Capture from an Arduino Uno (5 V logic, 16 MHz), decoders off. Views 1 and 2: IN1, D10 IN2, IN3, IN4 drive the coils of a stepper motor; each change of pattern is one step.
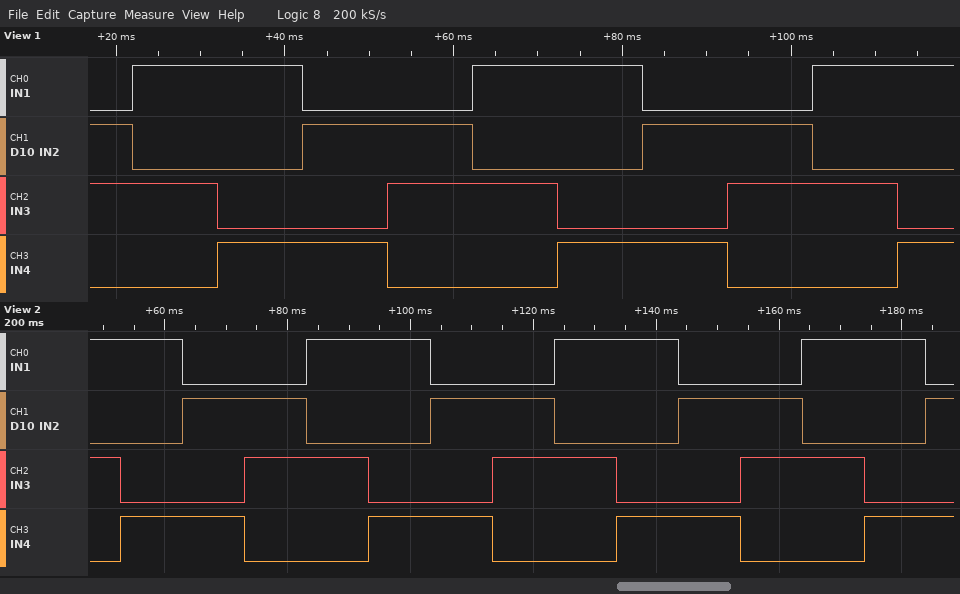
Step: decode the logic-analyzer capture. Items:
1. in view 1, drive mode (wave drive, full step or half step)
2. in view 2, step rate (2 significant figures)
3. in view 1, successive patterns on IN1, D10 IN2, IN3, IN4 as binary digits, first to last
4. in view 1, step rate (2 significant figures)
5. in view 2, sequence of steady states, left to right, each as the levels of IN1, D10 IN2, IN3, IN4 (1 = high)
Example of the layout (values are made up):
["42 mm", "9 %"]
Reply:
["full step", "99 steps/s", "0110 1010 1001 0101 0110 1010 1001 0101 0110 1010 1001", "99 steps/s", "1010 1001 0101 0110 1010 1001 0101 0110 1010 1001 0101 0110 1010 1001 0101"]
